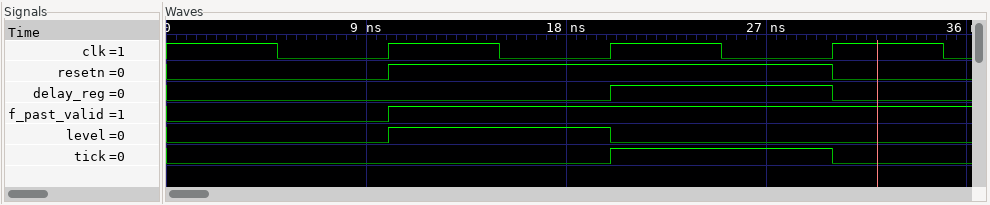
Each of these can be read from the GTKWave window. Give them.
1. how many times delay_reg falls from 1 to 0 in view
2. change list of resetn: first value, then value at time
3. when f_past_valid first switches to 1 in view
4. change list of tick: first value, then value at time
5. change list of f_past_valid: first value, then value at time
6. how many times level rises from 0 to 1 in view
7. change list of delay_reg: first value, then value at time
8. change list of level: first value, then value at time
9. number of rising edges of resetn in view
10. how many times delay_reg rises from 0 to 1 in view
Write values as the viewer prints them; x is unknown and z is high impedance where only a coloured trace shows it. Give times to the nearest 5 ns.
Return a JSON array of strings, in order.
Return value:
["1", "0, 1 at 10 ns, 0 at 30 ns", "10 ns", "0, 1 at 20 ns, 0 at 30 ns", "0, 1 at 10 ns", "1", "0, 1 at 20 ns, 0 at 30 ns", "0, 1 at 10 ns, 0 at 20 ns", "1", "1"]
